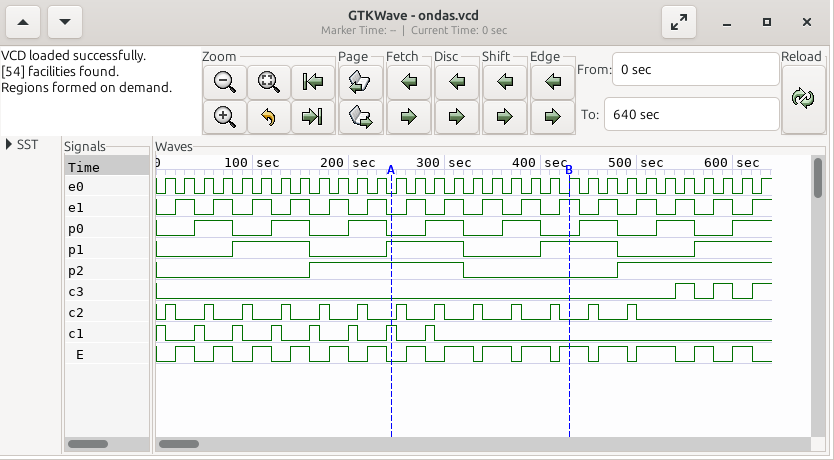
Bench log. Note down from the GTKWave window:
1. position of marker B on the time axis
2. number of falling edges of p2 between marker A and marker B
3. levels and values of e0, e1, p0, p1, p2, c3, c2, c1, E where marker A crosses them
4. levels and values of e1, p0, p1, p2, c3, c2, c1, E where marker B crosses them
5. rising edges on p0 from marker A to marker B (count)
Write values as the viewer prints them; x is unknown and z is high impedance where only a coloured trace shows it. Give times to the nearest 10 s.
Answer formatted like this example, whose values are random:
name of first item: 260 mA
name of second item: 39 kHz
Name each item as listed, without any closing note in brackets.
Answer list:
position of marker B on the time axis: 430 s
number of falling edges of p2 between marker A and marker B: 1
levels and values of e0, e1, p0, p1, p2, c3, c2, c1, E where marker A crosses them: e0=0, e1=0, p0=0, p1=1, p2=1, c3=0, c2=0, c1=1, E=0
levels and values of e1, p0, p1, p2, c3, c2, c1, E where marker B crosses them: e1=1, p0=0, p1=1, p2=0, c3=0, c2=0, c1=0, E=1
rising edges on p0 from marker A to marker B: 2
